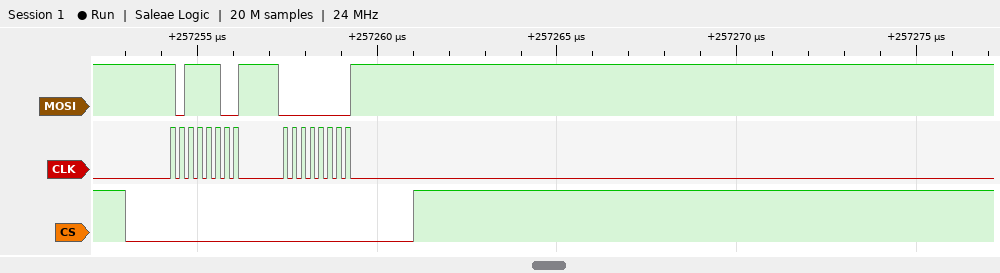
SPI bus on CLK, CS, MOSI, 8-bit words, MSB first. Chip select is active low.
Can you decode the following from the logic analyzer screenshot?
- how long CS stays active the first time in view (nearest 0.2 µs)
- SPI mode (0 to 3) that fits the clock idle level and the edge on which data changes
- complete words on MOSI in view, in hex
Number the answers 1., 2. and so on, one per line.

1. 8 µs
2. 0
3. BC, 00
